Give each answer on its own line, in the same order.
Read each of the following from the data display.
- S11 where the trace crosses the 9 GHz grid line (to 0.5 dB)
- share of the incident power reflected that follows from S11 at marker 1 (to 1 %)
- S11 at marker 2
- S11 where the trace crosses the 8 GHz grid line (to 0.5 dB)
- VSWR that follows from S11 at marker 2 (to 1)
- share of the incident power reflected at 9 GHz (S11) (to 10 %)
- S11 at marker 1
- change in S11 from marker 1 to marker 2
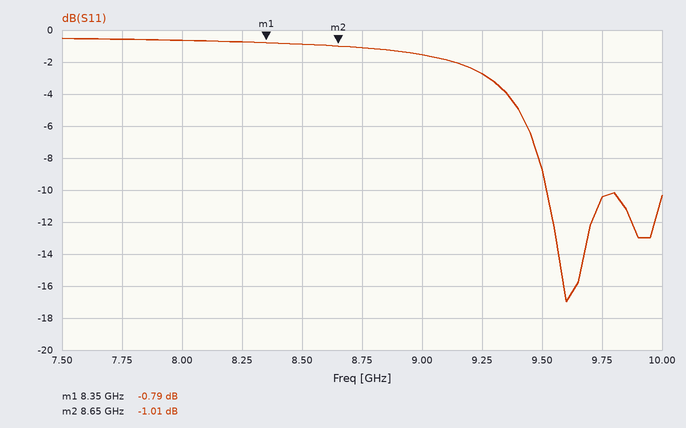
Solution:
-1.5 dB
83 %
-1.01 dB
-0.5 dB
17
70 %
-0.79 dB
-0.22 dB
